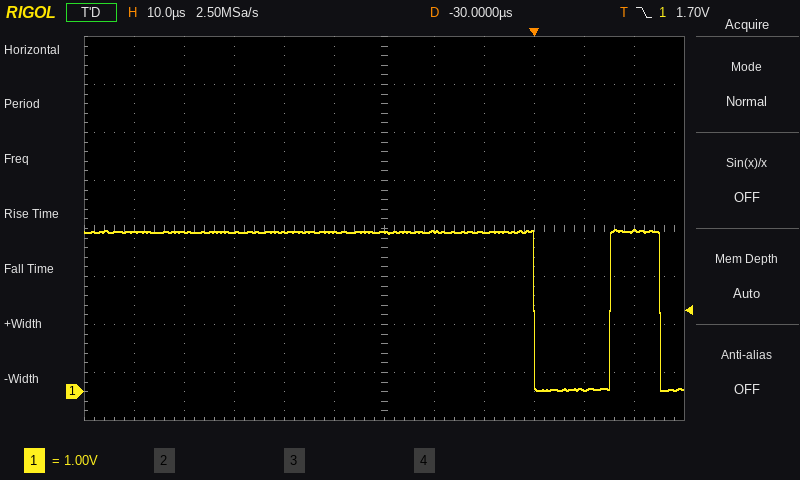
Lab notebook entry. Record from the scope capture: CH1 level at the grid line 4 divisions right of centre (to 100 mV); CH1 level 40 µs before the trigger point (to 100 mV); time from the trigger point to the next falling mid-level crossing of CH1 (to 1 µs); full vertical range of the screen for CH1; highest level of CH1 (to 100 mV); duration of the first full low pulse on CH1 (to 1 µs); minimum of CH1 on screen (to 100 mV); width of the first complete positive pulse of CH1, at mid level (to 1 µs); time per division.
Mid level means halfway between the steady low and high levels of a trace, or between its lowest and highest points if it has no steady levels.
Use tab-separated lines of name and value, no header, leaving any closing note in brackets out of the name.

CH1 level at the grid line 4 divisions right of centre	0.0 V
CH1 level 40 µs before the trigger point	3.3 V
time from the trigger point to the next falling mid-level crossing of CH1	25 µs
full vertical range of the screen for CH1	8 V
highest level of CH1	3.4 V
duration of the first full low pulse on CH1	15 µs
minimum of CH1 on screen	0.0 V
width of the first complete positive pulse of CH1, at mid level	10 µs
time per division	10 µs
